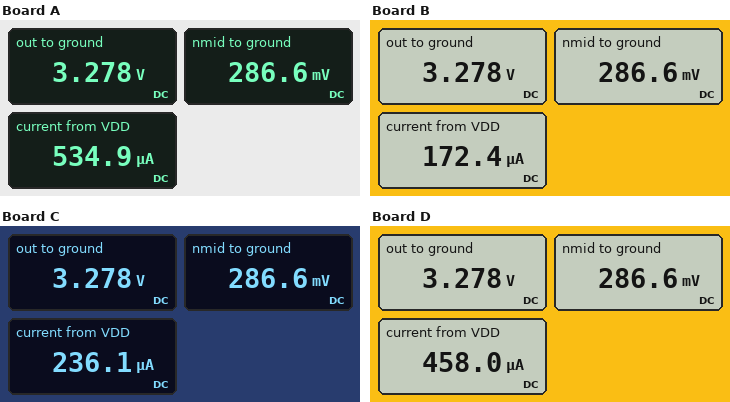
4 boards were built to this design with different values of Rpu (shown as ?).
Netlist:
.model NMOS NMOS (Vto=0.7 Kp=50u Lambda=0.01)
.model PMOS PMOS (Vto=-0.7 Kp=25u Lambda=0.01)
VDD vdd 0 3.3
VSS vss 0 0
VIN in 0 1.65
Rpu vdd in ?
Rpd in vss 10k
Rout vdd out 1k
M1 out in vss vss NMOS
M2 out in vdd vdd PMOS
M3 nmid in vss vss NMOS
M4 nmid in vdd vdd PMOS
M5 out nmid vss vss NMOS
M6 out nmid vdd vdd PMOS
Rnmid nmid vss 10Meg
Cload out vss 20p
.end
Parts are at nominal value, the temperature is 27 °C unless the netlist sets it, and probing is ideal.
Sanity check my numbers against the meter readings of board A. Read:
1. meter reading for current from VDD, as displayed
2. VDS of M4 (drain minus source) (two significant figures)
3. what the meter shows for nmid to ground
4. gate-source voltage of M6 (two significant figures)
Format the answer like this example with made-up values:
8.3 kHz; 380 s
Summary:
534.9 µA; -3.0 V; 286.6 mV; -3.0 V
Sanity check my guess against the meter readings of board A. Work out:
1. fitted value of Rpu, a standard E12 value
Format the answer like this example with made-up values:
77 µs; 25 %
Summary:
3.3 kΩ
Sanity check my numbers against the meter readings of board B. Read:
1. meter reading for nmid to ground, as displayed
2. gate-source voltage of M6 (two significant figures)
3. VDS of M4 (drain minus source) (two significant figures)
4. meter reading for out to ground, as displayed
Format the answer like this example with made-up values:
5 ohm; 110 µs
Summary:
286.6 mV; -3.0 V; -3.0 V; 3.278 V
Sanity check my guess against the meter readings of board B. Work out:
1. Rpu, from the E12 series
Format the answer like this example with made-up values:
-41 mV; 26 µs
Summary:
12 kΩ
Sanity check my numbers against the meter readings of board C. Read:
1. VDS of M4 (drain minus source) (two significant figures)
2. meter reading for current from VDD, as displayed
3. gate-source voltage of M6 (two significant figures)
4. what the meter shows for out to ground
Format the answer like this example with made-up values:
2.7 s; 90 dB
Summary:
-3.0 V; 236.1 µA; -3.0 V; 3.278 V
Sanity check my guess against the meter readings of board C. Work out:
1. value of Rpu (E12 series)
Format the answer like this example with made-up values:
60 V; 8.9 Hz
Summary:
8.2 kΩ
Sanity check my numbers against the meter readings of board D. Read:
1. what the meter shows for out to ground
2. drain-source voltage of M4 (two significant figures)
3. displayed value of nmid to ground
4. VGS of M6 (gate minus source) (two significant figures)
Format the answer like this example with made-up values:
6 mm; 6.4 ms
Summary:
3.278 V; -3.0 V; 286.6 mV; -3.0 V
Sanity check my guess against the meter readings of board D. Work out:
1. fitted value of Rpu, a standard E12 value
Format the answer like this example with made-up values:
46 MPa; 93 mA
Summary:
3.9 kΩ
